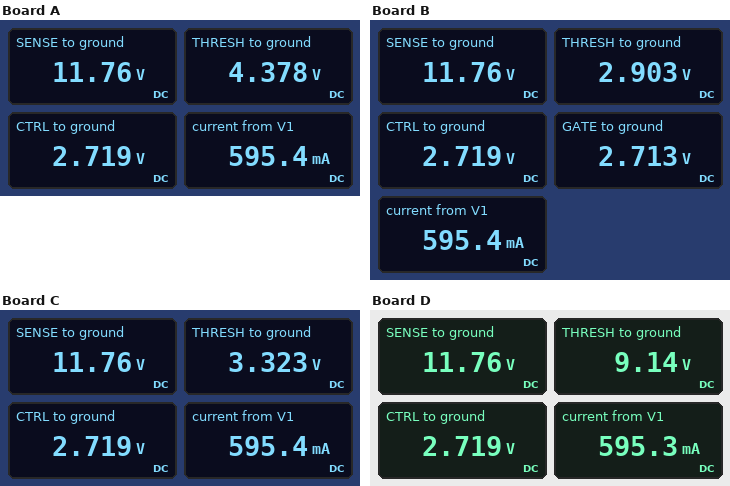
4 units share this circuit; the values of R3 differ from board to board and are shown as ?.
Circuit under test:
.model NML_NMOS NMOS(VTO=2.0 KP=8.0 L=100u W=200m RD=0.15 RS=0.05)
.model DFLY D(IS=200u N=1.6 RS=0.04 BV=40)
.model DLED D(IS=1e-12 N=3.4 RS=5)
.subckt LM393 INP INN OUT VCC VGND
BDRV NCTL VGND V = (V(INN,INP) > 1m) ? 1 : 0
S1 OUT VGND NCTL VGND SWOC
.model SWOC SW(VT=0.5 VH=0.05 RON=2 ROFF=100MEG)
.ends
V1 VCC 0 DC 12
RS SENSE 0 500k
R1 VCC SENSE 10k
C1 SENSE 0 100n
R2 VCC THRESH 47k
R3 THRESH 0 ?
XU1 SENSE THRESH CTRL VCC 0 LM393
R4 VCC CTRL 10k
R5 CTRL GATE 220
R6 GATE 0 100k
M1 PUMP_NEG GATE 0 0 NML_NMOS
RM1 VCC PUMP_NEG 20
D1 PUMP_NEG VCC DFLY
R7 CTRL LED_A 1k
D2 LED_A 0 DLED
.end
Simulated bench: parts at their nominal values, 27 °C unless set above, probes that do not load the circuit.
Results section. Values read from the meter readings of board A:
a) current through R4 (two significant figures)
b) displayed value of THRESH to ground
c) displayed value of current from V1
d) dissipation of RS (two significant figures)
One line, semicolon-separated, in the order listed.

930 µA; 4.378 V; 595.4 mA; 280 µW
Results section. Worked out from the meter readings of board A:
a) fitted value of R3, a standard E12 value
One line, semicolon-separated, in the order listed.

27 kΩ
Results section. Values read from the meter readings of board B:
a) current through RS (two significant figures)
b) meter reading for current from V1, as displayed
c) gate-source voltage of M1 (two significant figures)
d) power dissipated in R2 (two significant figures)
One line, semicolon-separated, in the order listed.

24 µA; 595.4 mA; 2.7 V; 1.8 mW
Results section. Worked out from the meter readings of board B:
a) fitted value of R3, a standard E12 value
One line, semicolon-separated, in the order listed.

15 kΩ
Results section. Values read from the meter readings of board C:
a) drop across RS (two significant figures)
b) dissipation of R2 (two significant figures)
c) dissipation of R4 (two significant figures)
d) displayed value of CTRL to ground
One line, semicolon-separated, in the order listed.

12 V; 1.6 mW; 8.6 mW; 2.719 V
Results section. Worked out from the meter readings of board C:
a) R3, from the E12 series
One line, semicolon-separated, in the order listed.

18 kΩ
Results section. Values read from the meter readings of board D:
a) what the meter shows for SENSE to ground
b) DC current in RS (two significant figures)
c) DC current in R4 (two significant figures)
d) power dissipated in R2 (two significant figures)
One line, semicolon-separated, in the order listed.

11.76 V; 24 µA; 930 µA; 170 µW
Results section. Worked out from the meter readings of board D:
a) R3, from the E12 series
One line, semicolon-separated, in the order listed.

150 kΩ
